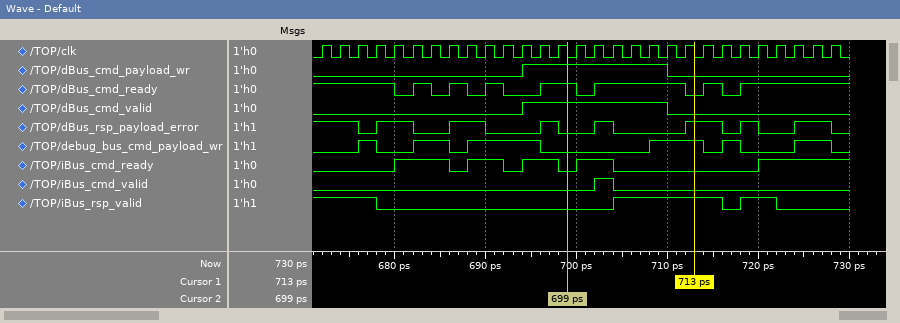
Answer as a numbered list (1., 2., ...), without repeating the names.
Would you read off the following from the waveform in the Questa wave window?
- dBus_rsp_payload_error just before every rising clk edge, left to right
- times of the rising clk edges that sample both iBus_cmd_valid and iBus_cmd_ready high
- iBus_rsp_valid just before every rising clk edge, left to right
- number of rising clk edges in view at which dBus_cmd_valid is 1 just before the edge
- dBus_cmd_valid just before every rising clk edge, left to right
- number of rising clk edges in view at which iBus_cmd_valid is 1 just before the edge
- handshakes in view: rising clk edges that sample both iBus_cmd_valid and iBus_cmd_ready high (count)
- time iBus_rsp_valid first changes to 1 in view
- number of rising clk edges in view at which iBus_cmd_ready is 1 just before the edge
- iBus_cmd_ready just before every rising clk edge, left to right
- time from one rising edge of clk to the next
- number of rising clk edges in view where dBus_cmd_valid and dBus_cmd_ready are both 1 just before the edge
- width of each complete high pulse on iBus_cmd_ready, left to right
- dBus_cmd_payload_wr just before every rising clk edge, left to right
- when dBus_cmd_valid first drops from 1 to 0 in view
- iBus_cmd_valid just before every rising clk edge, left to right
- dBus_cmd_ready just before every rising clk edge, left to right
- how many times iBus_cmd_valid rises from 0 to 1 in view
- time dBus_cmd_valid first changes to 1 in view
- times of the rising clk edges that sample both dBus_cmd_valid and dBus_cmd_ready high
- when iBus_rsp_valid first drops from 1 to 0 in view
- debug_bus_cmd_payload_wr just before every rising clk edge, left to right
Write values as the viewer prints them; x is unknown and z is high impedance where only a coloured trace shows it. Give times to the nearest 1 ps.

1. 1 1 1 0 1 1 0 0 1 1 0 0 0 1 0 0 1 0 0 0 0 1 1 0 1 0 0 1 1
2. 704 ps
3. 1 1 1 1 0 0 0 0 0 0 0 0 0 0 0 0 0 1 1 1 1 1 1 0 1 1 0 0 0
4. 8
5. 0 0 0 0 0 0 0 0 0 0 0 0 1 1 1 1 1 1 1 1 0 0 0 0 0 0 0 0 0
6. 1
7. 1
8. 704 ps
9. 13
10. 0 0 0 0 0 1 1 1 0 1 1 0 1 1 0 1 1 0 0 0 0 0 0 0 0 1 1 1 1
11. 2 ps
12. 6
13. 6 ps, 4 ps, 4 ps, 4 ps
14. 0 0 0 0 0 0 0 0 0 0 0 0 1 1 1 1 1 1 1 1 0 0 0 0 0 0 0 0 0
15. 710 ps
16. 0 0 0 0 0 0 0 0 0 0 0 0 0 0 0 0 1 0 0 0 0 0 0 0 0 0 0 0 0
17. 1 1 1 1 1 0 1 0 1 0 1 0 0 1 1 0 1 1 1 1 1 0 1 0 1 1 1 1 1
18. 1
19. 694 ps
20. 698 ps, 700 ps, 704 ps, 706 ps, 708 ps, 710 ps
21. 678 ps
22. 0 0 0 1 0 0 1 1 0 1 1 1 1 0 0 0 0 0 0 1 1 1 0 1 0 0 0 1 1
